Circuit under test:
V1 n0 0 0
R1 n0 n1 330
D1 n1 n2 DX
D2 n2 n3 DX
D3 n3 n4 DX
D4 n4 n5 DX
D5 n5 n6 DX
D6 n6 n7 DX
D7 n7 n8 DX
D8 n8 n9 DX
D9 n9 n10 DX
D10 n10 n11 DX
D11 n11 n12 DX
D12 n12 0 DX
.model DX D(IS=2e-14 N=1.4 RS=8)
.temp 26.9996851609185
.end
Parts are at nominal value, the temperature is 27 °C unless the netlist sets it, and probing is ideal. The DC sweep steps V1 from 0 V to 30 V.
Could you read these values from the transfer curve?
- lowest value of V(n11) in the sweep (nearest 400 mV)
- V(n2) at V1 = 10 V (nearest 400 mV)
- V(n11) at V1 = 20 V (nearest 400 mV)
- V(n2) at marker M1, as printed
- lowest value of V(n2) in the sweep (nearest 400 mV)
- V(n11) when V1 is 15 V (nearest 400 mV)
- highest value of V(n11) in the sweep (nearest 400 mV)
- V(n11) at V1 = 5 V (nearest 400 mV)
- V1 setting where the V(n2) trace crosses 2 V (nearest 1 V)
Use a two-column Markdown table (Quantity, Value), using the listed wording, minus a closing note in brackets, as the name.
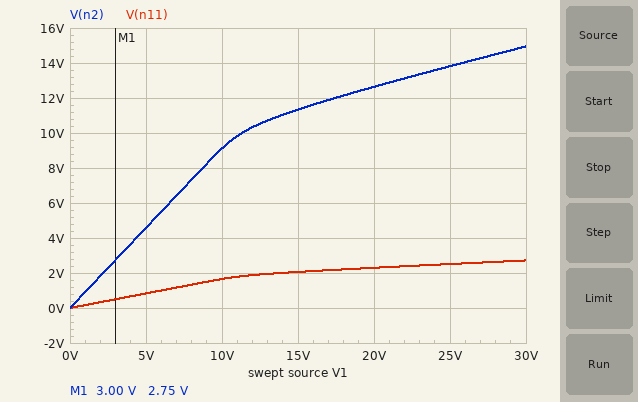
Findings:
| Quantity | Value |
|---|---|
| lowest value of V(n11) in the sweep | 0 V |
| V(n2) at V1 = 10 V | 9.2 V |
| V(n11) at V1 = 20 V | 2.4 V |
| V(n2) at marker M1, as printed | 2.75 V |
| lowest value of V(n2) in the sweep | 0 V |
| V(n11) when V1 is 15 V | 2.0 V |
| highest value of V(n11) in the sweep | 2.8 V |
| V(n11) at V1 = 5 V | 800 mV |
| V1 setting where the V(n2) trace crosses 2 V | 2 V |
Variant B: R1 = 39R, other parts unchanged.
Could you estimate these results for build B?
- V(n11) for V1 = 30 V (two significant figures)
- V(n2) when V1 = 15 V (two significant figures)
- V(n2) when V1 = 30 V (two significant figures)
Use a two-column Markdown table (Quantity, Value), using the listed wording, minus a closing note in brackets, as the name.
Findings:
| Quantity | Value |
|---|---|
| V(n11) for V1 = 30 V | 4.2 V |
| V(n2) when V1 = 15 V | 13 V |
| V(n2) when V1 = 30 V | 23 V |
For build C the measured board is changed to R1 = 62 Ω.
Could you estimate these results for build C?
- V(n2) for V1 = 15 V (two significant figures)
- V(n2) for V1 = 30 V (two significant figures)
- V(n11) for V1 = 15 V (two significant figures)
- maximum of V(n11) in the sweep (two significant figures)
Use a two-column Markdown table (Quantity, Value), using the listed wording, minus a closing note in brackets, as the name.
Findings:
| Quantity | Value |
|---|---|
| V(n2) for V1 = 15 V | 13 V |
| V(n2) for V1 = 30 V | 21 V |
| V(n11) for V1 = 15 V | 2.3 V |
| maximum of V(n11) in the sweep | 3.9 V |
